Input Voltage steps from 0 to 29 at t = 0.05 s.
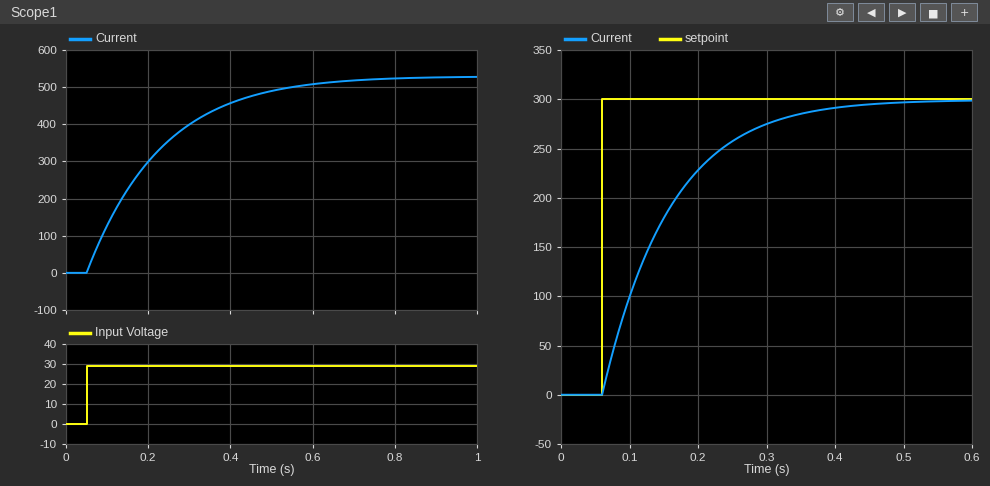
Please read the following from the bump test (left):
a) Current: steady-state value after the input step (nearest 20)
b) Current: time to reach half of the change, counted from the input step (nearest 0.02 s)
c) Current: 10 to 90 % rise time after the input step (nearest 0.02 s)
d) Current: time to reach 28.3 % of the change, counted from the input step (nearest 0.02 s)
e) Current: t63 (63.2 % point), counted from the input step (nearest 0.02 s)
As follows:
520
0.12 s
0.38 s
0.06 s
0.18 s
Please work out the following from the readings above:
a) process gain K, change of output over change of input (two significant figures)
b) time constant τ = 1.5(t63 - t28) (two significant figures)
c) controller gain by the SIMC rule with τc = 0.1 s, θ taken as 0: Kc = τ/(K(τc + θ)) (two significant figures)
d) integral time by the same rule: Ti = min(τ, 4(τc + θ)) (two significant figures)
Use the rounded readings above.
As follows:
18
0.18 s
0.10
0.18 s
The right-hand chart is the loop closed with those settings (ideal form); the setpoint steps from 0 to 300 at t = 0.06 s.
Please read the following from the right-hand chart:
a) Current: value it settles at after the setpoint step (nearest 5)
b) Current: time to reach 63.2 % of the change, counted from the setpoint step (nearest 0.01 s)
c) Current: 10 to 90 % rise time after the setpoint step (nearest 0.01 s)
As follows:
300
0.10 s
0.21 s
